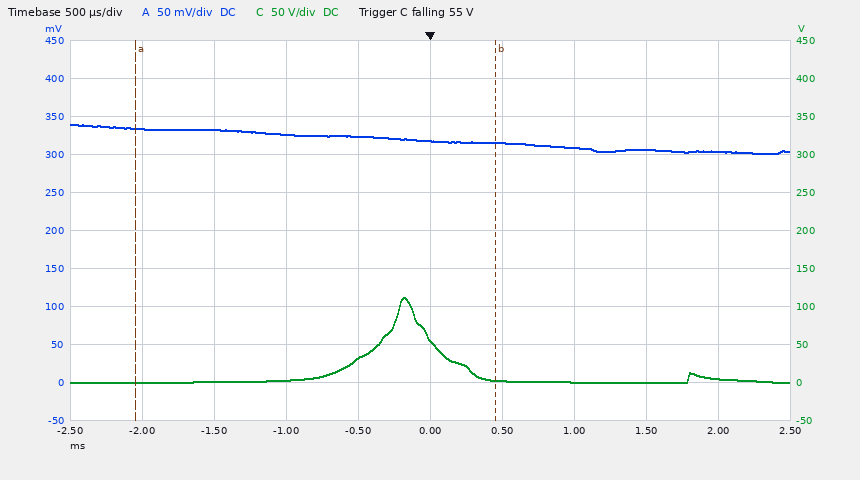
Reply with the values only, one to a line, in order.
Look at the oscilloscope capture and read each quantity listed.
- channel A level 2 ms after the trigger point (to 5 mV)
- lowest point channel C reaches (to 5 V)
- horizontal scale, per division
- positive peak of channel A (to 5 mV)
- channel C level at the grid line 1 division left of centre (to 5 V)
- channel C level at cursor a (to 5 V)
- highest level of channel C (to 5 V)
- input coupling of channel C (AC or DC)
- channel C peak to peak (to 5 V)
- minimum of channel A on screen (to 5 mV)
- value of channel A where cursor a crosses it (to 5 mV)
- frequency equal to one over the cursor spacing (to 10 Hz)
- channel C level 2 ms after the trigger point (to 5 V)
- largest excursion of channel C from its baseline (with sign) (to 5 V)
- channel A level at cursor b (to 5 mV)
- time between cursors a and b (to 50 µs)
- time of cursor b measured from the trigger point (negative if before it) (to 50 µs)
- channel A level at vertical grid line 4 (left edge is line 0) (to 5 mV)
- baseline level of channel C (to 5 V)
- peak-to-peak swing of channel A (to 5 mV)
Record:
305 mV
0 V
500 µs
340 mV
30 V
0 V
110 V
DC
110 V
300 mV
335 mV
400 Hz
5 V
+110 V
315 mV
2.50 ms
+450 µs
325 mV
0 V
40 mV
